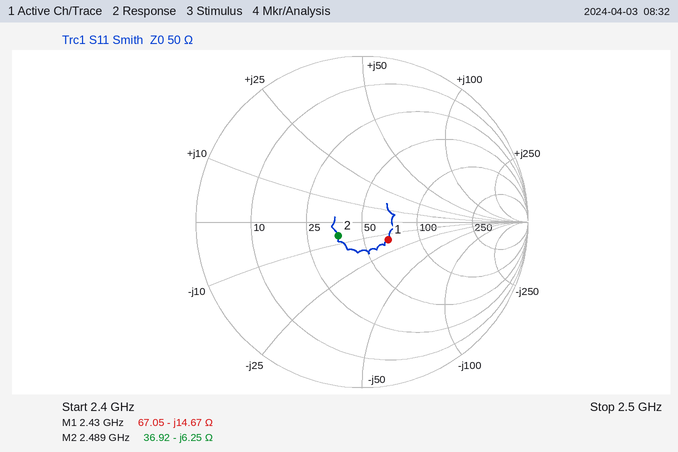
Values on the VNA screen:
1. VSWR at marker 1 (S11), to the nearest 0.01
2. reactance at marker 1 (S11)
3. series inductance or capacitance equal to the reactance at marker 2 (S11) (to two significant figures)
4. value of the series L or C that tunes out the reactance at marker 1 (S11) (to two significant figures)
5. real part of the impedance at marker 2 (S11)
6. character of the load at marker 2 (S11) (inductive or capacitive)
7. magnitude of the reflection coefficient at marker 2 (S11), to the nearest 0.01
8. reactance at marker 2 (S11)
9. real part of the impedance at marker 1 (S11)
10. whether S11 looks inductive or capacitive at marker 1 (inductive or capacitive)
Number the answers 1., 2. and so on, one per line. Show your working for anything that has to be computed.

1. 1.47
2. -14.67 Ω
3. C = 1/(2π × 2.489 GHz × 6.25 Ω) ≈ 10 pF
4. L = 14.67 Ω/(2π × 2.43 GHz) ≈ 961 pH, so 960 pH to two significant figures
5. 36.92 Ω
6. capacitive
7. 0.17
8. -6.25 Ω
9. 67.05 Ω
10. capacitive
